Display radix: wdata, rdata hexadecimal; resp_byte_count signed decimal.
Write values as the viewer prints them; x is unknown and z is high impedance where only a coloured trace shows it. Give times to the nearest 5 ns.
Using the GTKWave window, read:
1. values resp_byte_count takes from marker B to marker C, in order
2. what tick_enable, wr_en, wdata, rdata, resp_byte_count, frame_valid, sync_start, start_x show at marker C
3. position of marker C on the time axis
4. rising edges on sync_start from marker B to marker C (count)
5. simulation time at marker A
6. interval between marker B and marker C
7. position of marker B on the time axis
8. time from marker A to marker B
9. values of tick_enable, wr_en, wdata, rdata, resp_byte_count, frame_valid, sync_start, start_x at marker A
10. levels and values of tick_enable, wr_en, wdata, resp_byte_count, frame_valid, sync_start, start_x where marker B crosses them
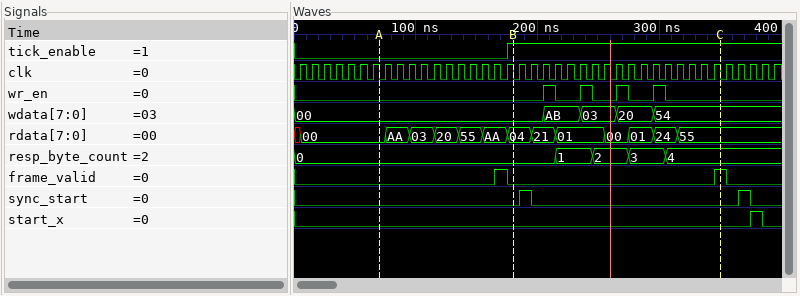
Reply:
0, 1, 2, 3, 4
tick_enable=1, wr_en=0, wdata=54, rdata=55, resp_byte_count=4, frame_valid=1, sync_start=0, start_x=0
350 ns
1
70 ns
170 ns
180 ns
110 ns
tick_enable=0, wr_en=0, wdata=00, rdata=00, resp_byte_count=0, frame_valid=0, sync_start=0, start_x=0
tick_enable=1, wr_en=0, wdata=00, resp_byte_count=0, frame_valid=0, sync_start=0, start_x=0
